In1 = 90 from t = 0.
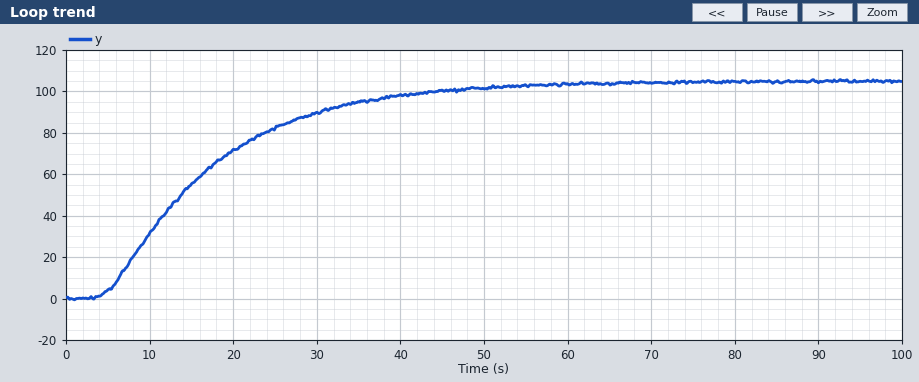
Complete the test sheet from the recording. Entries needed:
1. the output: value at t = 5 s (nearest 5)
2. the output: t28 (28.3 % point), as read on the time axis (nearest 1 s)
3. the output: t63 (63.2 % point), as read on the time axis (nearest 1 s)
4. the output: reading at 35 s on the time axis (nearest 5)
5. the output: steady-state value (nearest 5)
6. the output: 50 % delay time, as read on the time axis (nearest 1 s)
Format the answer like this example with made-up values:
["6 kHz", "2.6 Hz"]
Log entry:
["5", "10 s", "18 s", "95", "105", "14 s"]
